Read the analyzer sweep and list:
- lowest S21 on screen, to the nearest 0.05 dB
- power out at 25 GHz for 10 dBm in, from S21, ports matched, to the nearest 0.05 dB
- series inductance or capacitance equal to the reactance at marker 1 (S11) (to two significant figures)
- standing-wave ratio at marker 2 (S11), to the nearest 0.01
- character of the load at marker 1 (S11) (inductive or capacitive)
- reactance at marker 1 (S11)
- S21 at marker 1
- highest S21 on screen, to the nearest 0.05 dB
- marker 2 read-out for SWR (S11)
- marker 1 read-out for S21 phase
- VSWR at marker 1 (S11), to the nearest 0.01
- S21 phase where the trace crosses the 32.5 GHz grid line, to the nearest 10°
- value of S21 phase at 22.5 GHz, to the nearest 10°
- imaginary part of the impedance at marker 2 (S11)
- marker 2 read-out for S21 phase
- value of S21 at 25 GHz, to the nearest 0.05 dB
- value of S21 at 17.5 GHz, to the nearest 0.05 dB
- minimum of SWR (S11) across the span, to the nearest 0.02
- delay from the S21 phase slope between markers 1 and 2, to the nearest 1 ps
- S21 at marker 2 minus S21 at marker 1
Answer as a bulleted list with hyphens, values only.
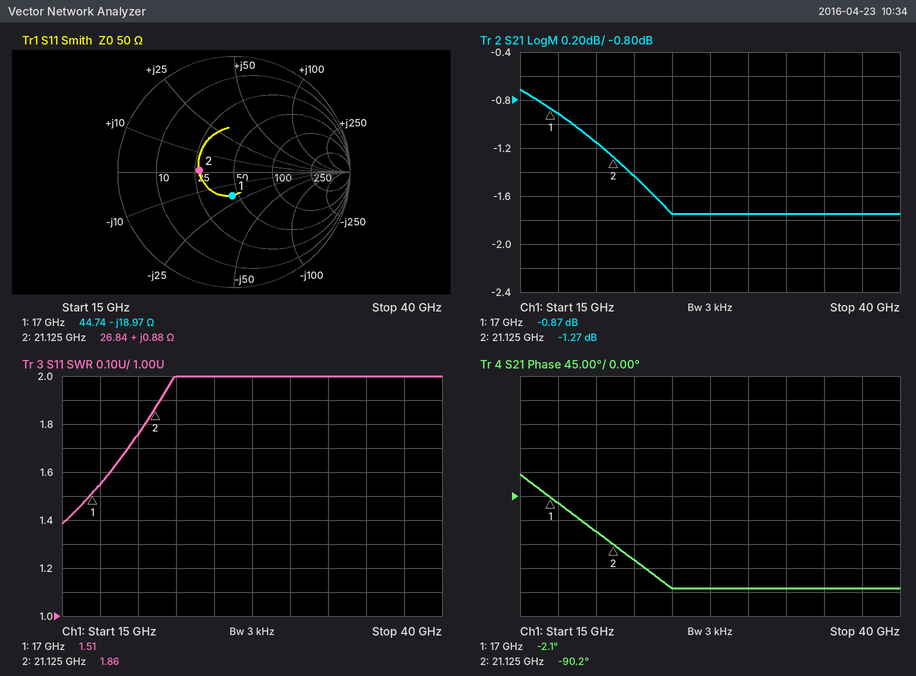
- -1.75 dB
- 8.25 dBm
- 490 fF
- 1.86
- capacitive
- -18.97 Ω
- -0.87 dB
- -0.70 dB
- 1.86
- -2.1°
- 1.51
- -170°
- -120°
- +0.88 Ω
- -90.2°
- -1.75 dB
- -0.90 dB
- 1.38
- 59 ps
- -0.40 dB
